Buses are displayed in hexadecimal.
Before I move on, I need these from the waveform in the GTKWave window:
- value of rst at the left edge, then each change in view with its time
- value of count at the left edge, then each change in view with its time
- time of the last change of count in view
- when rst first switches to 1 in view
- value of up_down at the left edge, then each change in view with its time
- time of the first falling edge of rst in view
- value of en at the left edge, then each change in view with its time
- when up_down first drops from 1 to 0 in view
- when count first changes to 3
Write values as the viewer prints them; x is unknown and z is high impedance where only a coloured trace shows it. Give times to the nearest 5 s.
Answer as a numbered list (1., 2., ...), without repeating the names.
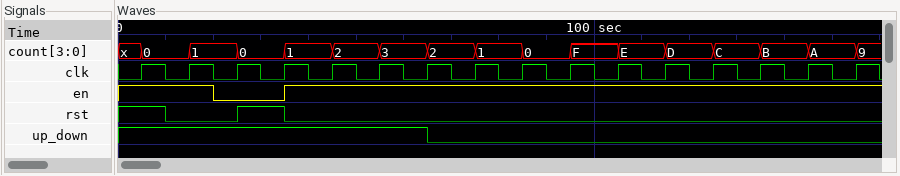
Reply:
1. 1, 0 at 10 s, 1 at 25 s, 0 at 35 s
2. x, 0 at 5 s, 1 at 15 s, 0 at 25 s, 1 at 35 s, 2 at 45 s, 3 at 55 s, 2 at 65 s, 1 at 75 s, 0 at 85 s, F at 95 s, E at 105 s, D at 115 s, C at 125 s, B at 135 s, A at 145 s, 9 at 155 s
3. 155 s
4. 25 s
5. 1, 0 at 65 s
6. 10 s
7. 1, 0 at 20 s, 1 at 35 s
8. 65 s
9. 55 s
